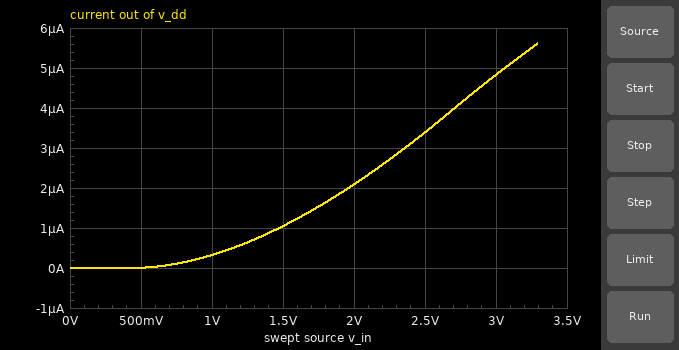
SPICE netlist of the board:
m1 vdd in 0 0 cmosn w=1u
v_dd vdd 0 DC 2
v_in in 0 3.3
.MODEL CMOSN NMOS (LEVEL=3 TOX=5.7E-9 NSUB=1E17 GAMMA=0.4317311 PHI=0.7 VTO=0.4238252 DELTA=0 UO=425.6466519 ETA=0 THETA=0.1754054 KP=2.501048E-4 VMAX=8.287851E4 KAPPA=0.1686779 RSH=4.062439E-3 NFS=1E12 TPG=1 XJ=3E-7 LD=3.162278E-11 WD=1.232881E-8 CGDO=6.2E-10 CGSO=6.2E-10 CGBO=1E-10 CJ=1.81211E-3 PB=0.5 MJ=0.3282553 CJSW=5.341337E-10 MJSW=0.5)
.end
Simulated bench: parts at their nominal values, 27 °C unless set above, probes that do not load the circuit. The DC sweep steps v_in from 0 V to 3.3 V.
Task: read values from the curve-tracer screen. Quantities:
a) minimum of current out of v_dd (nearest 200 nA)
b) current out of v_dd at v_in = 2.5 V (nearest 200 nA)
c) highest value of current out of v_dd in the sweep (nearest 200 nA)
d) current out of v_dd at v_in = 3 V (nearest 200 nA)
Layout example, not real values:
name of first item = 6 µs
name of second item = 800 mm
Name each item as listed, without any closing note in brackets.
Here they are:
minimum of current out of v_dd = 0 A
current out of v_dd at v_in = 2.5 V = 3.4 µA
highest value of current out of v_dd in the sweep = 5.6 µA
current out of v_dd at v_in = 3 V = 4.8 µA
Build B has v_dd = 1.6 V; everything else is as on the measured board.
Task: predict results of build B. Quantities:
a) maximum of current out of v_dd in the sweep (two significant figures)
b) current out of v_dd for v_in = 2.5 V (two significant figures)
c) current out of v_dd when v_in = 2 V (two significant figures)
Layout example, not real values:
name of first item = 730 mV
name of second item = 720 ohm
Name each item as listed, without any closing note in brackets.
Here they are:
maximum of current out of v_dd in the sweep = 5.1 µA
current out of v_dd for v_in = 2.5 V = 3.3 µA
current out of v_dd when v_in = 2 V = 2.1 µA
